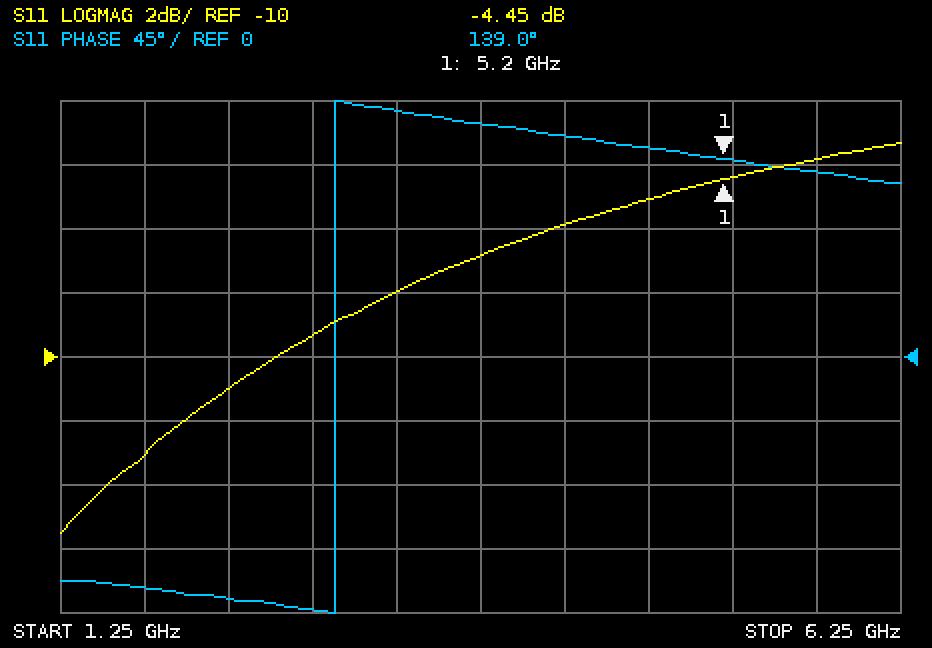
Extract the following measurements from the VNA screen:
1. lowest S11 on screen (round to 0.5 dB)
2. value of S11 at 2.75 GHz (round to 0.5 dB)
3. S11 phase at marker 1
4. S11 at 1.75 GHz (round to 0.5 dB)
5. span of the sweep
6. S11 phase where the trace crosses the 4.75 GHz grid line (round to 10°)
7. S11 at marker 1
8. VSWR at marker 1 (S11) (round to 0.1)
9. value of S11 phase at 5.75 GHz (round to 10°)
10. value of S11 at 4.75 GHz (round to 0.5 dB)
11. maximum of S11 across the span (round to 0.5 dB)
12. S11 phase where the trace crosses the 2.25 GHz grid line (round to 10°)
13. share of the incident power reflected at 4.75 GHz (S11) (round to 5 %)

-15.5 dB
-9.5 dB
139.0°
-13.0 dB
5 GHz
150°
-4.45 dB
4.0
130°
-5.0 dB
-3.5 dB
-170°
30 %
